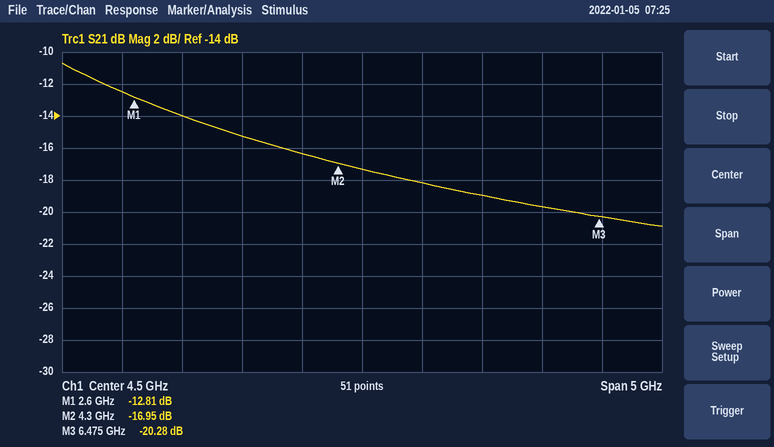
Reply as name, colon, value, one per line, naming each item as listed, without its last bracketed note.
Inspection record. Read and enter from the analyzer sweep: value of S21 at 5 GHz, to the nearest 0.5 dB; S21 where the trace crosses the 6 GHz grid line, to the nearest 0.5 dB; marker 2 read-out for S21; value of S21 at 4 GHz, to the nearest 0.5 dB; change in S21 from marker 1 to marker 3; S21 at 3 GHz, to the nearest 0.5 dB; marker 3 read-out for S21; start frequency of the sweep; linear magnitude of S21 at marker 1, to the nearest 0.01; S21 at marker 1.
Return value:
value of S21 at 5 GHz, to the nearest 0.5 dB: -18.0 dB
S21 where the trace crosses the 6 GHz grid line, to the nearest 0.5 dB: -19.5 dB
marker 2 read-out for S21: -16.95 dB
value of S21 at 4 GHz, to the nearest 0.5 dB: -16.5 dB
change in S21 from marker 1 to marker 3: -7.47 dB
S21 at 3 GHz, to the nearest 0.5 dB: -14.0 dB
marker 3 read-out for S21: -20.28 dB
start frequency of the sweep: 2 GHz
linear magnitude of S21 at marker 1, to the nearest 0.01: 0.23
S21 at marker 1: -12.81 dB
